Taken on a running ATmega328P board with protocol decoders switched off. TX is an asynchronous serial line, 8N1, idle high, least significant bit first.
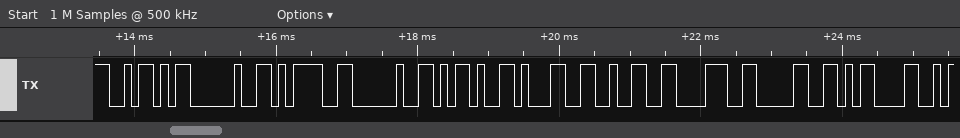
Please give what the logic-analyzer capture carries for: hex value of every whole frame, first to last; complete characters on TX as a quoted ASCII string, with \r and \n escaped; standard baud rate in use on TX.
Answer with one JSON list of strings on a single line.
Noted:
["5A 20 3D 20 2D 31 32 38 30 0D", "\"Z = -1280\\r\"", "9600 baud"]
